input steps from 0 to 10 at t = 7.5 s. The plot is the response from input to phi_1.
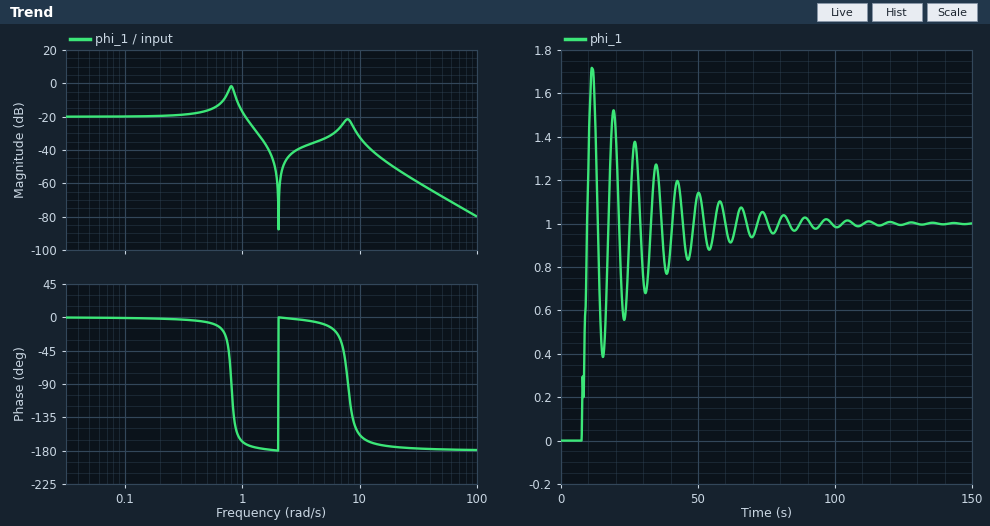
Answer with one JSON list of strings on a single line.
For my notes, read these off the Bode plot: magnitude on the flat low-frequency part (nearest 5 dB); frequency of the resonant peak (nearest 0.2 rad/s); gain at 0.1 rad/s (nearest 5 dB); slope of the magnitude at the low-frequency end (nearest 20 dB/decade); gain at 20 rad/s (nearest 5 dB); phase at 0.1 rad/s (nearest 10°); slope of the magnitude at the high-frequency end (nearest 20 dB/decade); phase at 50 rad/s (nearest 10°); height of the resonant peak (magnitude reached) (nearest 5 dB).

["-20 dB", "0.8 rad/s", "-20 dB", "0 dB/decade", "-50 dB", "0°", "-40 dB/decade", "-180°", "0 dB"]
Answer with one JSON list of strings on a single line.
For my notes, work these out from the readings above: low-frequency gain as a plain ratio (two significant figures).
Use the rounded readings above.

["0.10"]
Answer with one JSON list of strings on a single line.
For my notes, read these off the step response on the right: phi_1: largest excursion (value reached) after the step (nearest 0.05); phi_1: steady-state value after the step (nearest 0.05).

["1.70", "1.00"]
